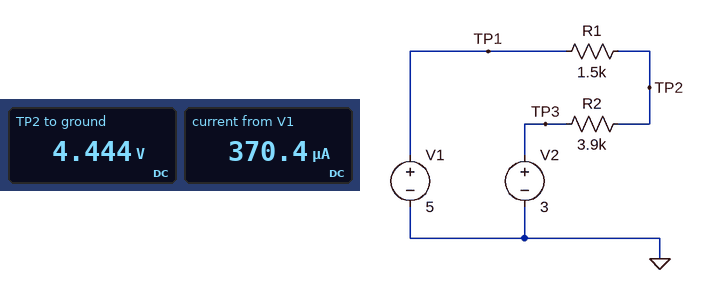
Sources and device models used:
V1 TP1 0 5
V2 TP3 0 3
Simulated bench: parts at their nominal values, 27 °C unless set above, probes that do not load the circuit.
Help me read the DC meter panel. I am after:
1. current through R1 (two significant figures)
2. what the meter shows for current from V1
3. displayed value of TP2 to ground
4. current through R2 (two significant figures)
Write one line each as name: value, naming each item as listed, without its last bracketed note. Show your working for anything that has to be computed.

current through R1: (5 V - 4.444 V) / 1.5 kΩ = 370 µA
what the meter shows for current from V1: 370.4 µA
displayed value of TP2 to ground: 4.444 V
current through R2: (4.444 V - 3 V) / 3.9 kΩ = 370 µA
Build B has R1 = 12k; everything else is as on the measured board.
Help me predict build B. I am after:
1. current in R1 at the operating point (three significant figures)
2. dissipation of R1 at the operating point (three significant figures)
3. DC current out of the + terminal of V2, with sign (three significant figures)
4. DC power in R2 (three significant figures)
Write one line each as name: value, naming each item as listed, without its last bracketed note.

current in R1 at the operating point: 126 µA
dissipation of R1 at the operating point: 190 µW
DC current out of the + terminal of V2, with sign: -126 µA
DC power in R2: 61.7 µW
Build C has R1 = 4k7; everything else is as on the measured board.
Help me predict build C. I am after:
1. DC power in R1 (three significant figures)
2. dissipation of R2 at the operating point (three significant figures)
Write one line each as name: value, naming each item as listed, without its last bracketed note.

DC power in R1: 254 µW
dissipation of R2 at the operating point: 211 µW
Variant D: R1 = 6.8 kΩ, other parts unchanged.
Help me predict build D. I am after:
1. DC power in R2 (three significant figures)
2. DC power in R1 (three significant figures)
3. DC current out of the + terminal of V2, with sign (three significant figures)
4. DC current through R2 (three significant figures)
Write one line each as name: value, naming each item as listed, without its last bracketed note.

DC power in R2: 136 µW
DC power in R1: 238 µW
DC current out of the + terminal of V2, with sign: -187 µA
DC current through R2: 187 µA
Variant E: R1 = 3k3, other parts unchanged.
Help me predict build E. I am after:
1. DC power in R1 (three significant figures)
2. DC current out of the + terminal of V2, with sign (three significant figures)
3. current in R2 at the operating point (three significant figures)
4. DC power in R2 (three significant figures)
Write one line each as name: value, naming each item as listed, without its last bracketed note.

DC power in R1: 255 µW
DC current out of the + terminal of V2, with sign: -278 µA
current in R2 at the operating point: 278 µA
DC power in R2: 301 µW
